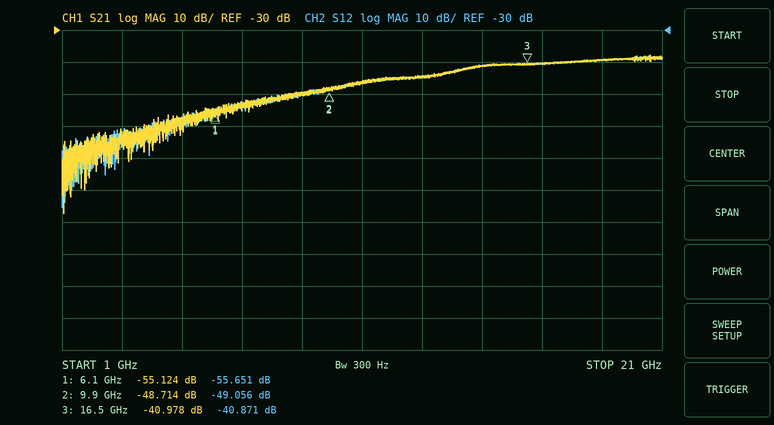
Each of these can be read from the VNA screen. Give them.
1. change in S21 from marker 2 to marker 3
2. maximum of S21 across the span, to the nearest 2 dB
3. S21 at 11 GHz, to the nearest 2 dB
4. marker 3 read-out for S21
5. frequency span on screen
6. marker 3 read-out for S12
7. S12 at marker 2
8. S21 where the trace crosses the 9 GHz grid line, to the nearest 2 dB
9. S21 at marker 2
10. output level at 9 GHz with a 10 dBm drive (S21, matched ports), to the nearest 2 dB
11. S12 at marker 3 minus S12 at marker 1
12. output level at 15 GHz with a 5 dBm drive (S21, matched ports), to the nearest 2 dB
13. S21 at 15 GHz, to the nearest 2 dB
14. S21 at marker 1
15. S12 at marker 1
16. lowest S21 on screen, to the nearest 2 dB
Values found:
7.736 dB
-38 dB
-46 dB
-40.978 dB
20 GHz
-40.871 dB
-49.056 dB
-50 dB
-48.714 dB
-40 dBm
14.780 dB
-36 dBm
-42 dB
-55.124 dB
-55.651 dB
-88 dB
